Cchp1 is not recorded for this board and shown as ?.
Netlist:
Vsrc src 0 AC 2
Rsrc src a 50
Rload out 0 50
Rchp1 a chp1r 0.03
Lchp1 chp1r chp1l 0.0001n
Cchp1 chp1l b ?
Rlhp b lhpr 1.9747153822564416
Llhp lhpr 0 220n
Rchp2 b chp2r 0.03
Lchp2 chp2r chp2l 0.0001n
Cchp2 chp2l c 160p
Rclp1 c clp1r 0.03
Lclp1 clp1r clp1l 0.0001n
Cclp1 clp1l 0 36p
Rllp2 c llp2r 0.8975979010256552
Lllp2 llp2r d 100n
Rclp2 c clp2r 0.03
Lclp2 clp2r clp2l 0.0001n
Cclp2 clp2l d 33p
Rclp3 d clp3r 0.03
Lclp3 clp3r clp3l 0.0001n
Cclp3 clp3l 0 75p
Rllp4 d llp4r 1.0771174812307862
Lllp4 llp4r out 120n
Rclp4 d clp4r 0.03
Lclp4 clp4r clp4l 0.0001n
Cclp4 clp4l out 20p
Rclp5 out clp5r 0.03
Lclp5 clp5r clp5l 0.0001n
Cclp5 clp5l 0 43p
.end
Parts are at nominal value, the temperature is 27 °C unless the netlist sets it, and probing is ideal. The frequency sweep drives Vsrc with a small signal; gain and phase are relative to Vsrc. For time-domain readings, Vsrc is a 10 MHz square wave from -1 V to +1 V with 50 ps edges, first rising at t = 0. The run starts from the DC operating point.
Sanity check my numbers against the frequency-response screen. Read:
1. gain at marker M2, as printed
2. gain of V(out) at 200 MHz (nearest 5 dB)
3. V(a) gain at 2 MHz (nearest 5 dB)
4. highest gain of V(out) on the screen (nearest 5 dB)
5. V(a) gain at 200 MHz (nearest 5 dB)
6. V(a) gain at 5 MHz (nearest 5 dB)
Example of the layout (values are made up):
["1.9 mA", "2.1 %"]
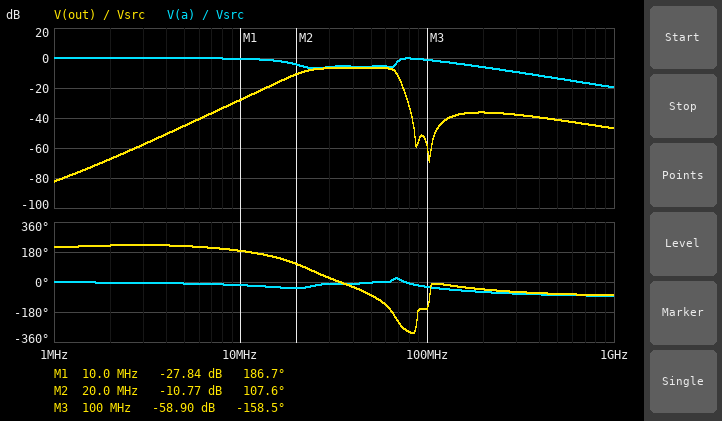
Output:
["-10.77 dB", "-35 dB", "0 dB", "-5 dB", "-5 dB", "0 dB"]
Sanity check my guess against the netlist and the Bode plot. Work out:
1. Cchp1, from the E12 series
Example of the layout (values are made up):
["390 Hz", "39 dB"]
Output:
["100 pF"]
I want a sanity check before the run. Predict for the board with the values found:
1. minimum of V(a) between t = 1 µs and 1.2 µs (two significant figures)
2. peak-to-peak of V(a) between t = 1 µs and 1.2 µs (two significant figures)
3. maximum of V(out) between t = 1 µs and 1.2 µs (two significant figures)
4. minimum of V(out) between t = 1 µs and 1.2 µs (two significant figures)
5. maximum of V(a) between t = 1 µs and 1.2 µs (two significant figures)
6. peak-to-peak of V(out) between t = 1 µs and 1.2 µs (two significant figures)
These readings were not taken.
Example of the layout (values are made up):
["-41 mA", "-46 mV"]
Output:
["-1.1 V", "2.2 V", "380 mV", "-380 mV", "1.1 V", "760 mV"]
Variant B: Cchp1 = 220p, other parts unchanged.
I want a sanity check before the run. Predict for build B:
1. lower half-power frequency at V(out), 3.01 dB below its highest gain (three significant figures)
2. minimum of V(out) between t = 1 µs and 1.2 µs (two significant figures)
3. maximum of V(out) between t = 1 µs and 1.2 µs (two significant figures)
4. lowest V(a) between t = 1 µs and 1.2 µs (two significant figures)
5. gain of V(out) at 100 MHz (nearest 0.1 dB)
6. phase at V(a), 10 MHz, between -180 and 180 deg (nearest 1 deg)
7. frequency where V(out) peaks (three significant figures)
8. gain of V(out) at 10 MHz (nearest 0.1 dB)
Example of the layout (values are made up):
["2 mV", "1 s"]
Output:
["19.2 MHz", "-400 mV", "400 mV", "-1.1 V", "-58.2 dB", "-40 deg", "39.7 MHz", "-22.0 dB"]
